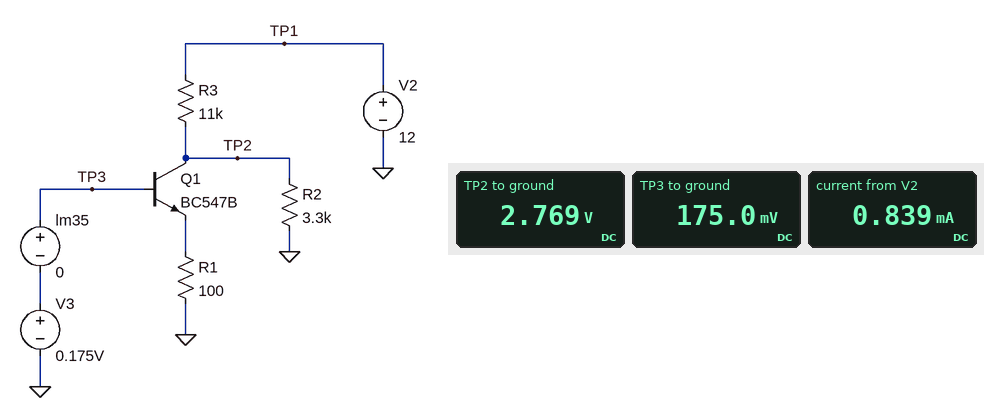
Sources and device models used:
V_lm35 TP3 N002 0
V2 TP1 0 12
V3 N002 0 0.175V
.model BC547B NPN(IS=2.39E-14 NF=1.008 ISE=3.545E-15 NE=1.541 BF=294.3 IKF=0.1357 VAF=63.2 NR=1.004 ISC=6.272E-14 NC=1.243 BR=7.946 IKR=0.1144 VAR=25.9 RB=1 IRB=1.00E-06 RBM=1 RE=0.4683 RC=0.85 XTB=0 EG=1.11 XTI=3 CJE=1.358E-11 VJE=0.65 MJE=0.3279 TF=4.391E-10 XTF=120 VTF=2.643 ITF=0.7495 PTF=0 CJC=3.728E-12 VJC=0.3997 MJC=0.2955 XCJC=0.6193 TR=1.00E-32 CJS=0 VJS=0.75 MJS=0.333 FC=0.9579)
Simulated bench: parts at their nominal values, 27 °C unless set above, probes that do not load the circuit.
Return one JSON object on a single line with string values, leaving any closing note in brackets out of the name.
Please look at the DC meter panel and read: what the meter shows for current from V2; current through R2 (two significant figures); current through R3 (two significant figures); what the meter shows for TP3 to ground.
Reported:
{"what the meter shows for current from V2": "0.839 mA", "current through R2": "840 µA", "current through R3": "840 µA", "what the meter shows for TP3 to ground": "175.0 mV"}
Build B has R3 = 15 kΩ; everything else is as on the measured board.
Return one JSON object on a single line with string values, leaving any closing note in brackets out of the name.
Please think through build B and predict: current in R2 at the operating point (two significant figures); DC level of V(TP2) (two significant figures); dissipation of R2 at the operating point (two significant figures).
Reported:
{"current in R2 at the operating point": "660 µA", "DC level of V(TP2)": "2.2 V", "dissipation of R2 at the operating point": "1.4 mW"}
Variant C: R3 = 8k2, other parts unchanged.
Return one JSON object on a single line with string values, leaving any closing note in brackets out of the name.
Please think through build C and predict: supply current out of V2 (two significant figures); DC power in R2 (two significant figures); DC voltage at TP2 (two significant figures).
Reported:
{"supply current out of V2": "1.0 mA", "DC power in R2": "3.6 mW", "DC voltage at TP2": "3.4 V"}
